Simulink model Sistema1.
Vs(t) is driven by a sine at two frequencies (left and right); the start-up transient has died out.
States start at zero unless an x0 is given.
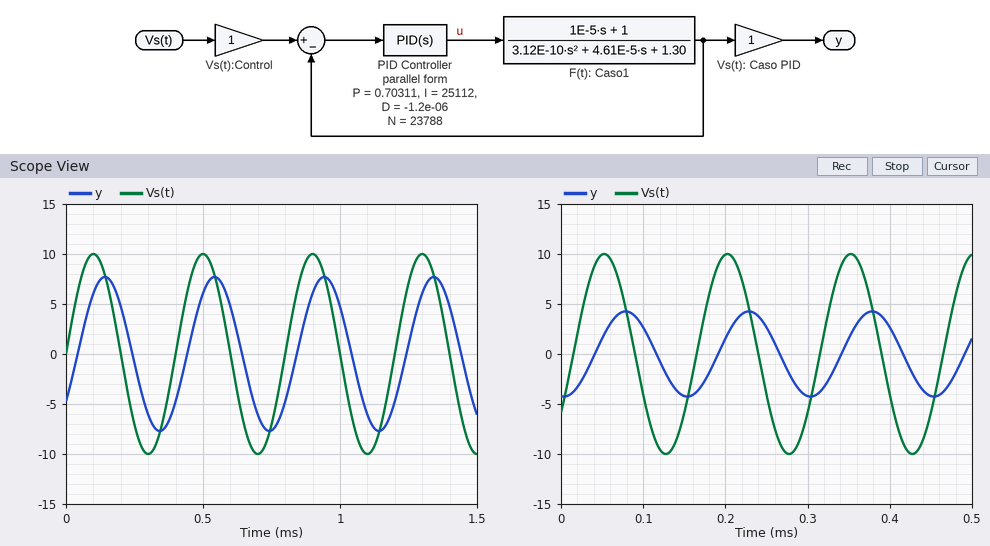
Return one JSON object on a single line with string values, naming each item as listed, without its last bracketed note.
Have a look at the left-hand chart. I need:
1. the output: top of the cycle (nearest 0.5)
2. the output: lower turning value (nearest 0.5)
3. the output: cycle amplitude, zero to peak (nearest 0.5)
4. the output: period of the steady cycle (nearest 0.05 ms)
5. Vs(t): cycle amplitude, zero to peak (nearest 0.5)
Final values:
{"the output: top of the cycle": "7.5", "the output: lower turning value": "-7.5", "the output: cycle amplitude, zero to peak": "7.5", "the output: period of the steady cycle": "0.40 ms", "Vs(t): cycle amplitude, zero to peak": "10.0"}
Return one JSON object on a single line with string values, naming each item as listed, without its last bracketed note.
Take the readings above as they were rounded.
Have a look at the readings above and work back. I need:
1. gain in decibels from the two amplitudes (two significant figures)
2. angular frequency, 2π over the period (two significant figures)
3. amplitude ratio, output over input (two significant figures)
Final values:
{"gain in decibels from the two amplitudes": "-2.5 dB", "angular frequency, 2π over the period": "16 rad/ms", "amplitude ratio, output over input": "0.75"}
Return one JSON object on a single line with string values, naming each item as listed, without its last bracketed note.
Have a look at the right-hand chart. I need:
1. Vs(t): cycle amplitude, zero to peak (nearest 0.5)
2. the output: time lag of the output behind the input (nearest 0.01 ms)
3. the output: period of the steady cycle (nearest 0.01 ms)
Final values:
{"Vs(t): cycle amplitude, zero to peak": "10.0", "the output: time lag of the output behind the input": "0.03 ms", "the output: period of the steady cycle": "0.15 ms"}
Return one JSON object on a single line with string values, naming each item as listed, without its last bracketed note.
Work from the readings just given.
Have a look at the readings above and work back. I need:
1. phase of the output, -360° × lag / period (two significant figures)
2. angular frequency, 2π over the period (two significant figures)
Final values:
{"phase of the output, -360° × lag / period": "-72°", "angular frequency, 2π over the period": "42 rad/ms"}
